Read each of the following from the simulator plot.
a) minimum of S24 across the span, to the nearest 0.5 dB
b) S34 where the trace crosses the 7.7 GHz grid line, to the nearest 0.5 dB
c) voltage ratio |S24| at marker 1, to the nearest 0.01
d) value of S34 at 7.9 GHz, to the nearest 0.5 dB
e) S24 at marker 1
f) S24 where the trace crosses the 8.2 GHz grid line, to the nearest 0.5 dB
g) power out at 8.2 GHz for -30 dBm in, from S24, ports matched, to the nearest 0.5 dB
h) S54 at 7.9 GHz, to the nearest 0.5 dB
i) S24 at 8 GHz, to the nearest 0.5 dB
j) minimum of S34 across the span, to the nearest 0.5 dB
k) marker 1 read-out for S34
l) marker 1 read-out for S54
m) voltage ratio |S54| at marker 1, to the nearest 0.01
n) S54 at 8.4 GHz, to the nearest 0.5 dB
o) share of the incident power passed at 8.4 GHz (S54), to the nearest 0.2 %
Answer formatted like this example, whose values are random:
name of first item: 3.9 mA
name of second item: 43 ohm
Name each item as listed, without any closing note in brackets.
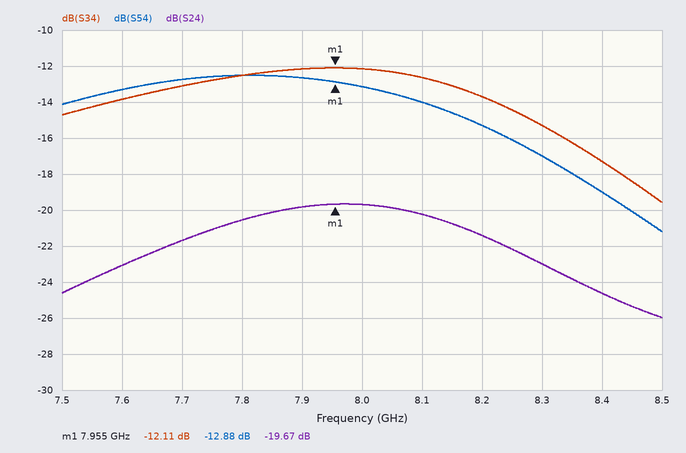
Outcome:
minimum of S24 across the span, to the nearest 0.5 dB: -26.0 dB
S34 where the trace crosses the 7.7 GHz grid line, to the nearest 0.5 dB: -13.0 dB
voltage ratio |S24| at marker 1, to the nearest 0.01: 0.10
value of S34 at 7.9 GHz, to the nearest 0.5 dB: -12.0 dB
S24 at marker 1: -19.67 dB
S24 where the trace crosses the 8.2 GHz grid line, to the nearest 0.5 dB: -21.5 dB
power out at 8.2 GHz for -30 dBm in, from S24, ports matched, to the nearest 0.5 dB: -51.5 dBm
S54 at 7.9 GHz, to the nearest 0.5 dB: -12.5 dB
S24 at 8 GHz, to the nearest 0.5 dB: -19.5 dB
minimum of S34 across the span, to the nearest 0.5 dB: -19.5 dB
marker 1 read-out for S34: -12.11 dB
marker 1 read-out for S54: -12.88 dB
voltage ratio |S54| at marker 1, to the nearest 0.01: 0.23
S54 at 8.4 GHz, to the nearest 0.5 dB: -19.0 dB
share of the incident power passed at 8.4 GHz (S54), to the nearest 0.2 %: 1.2 %
